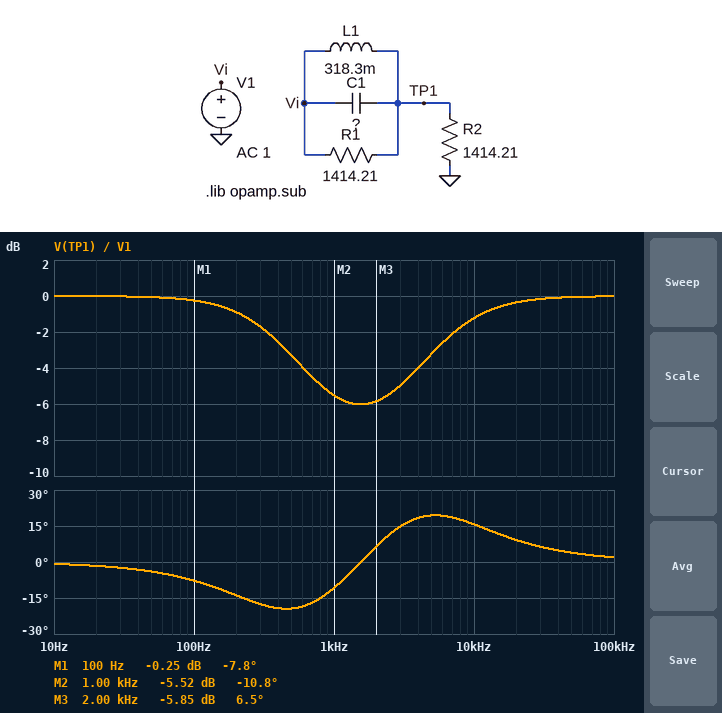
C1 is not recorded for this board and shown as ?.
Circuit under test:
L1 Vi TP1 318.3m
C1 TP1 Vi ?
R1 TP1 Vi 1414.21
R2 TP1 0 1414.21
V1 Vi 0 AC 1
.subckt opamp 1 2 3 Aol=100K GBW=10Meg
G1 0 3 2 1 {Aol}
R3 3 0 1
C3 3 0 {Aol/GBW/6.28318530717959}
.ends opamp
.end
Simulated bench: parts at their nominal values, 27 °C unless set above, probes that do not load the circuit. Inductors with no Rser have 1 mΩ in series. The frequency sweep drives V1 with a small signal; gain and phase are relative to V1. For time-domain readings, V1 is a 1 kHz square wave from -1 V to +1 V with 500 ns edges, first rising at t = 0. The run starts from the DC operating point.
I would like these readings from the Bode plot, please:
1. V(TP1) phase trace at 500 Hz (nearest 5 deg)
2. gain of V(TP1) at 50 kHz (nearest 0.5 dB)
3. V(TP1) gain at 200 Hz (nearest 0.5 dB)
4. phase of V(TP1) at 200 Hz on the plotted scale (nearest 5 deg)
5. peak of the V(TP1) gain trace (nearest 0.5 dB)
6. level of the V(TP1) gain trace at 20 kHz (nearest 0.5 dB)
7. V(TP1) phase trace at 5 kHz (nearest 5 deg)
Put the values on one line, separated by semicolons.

-20 deg; 0 dB; -1.0 dB; -15 deg; 0 dB; -0.5 dB; 20 deg
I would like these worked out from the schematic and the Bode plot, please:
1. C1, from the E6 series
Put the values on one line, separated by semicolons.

33 nF
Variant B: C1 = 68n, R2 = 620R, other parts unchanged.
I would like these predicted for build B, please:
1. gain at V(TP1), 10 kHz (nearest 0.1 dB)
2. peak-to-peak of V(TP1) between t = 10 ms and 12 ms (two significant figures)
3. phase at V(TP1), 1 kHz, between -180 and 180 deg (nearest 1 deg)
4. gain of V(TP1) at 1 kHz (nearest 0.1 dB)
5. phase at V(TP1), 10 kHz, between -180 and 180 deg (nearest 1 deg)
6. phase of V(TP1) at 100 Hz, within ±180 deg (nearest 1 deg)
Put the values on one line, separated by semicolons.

-1.0 dB; 3.0 V; -4 deg; -10.3 dB; 19 deg; -17 deg
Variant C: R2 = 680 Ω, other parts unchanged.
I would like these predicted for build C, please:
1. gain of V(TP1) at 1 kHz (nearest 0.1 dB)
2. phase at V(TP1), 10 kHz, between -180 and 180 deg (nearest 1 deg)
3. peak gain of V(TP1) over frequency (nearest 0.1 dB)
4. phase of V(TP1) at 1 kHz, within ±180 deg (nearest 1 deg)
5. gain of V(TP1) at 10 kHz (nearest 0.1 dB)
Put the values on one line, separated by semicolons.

-9.2 dB; 28 deg; 0 dB; -15 deg; -2.8 dB
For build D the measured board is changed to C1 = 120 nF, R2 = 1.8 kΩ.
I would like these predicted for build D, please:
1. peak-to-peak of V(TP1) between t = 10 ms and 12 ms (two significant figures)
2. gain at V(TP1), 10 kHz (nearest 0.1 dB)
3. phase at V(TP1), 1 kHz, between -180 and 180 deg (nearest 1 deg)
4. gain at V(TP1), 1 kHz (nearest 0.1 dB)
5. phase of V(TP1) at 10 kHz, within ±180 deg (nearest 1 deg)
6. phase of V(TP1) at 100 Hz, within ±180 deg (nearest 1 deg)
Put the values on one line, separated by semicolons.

2.6 V; -0.1 dB; 8 deg; -4.7 dB; 4 deg; -6 deg
